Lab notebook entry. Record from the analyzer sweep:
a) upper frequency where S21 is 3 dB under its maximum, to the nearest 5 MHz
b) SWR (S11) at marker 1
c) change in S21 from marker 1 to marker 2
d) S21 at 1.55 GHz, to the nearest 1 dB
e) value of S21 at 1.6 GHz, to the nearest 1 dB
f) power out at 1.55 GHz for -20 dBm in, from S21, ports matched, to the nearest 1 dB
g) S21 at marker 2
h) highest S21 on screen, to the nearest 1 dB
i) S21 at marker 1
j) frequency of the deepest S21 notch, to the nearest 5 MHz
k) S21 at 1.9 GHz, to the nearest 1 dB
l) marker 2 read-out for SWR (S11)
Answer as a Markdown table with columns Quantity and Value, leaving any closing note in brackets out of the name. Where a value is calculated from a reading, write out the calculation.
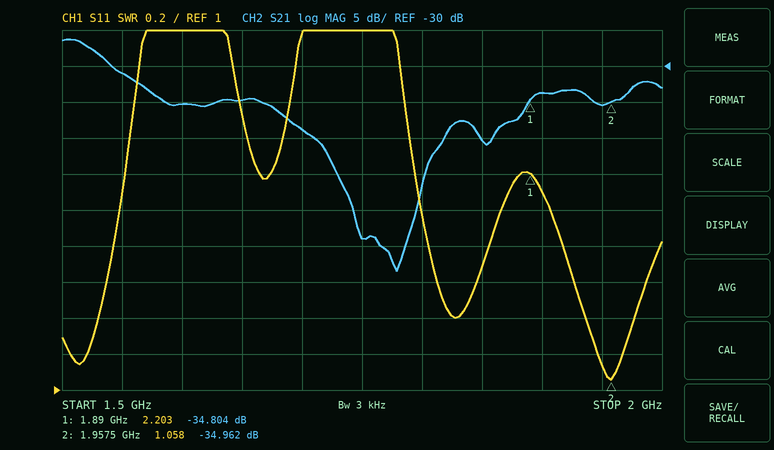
| Quantity | Value |
|---|---|
| upper frequency where S21 is 3 dB under its maximum, to the nearest 5 MHz | 1.535 GHz |
| SWR (S11) at marker 1 | 2.203 |
| change in S21 from marker 1 to marker 2 | -34.962 − (-34.804) = -0.158 dB |
| S21 at 1.55 GHz, to the nearest 1 dB | -31 dB |
| value of S21 at 1.6 GHz, to the nearest 1 dB | -35 dB |
| power out at 1.55 GHz for -20 dBm in, from S21, ports matched, to the nearest 1 dB | -20 dBm + (-31 dB) = -51 dBm |
| S21 at marker 2 | -34.962 dB |
| highest S21 on screen, to the nearest 1 dB | -26 dB |
| S21 at marker 1 | -34.804 dB |
| frequency of the deepest S21 notch, to the nearest 5 MHz | 1.780 GHz |
| S21 at 1.9 GHz, to the nearest 1 dB | -34 dB |
| marker 2 read-out for SWR | 1.058 |
